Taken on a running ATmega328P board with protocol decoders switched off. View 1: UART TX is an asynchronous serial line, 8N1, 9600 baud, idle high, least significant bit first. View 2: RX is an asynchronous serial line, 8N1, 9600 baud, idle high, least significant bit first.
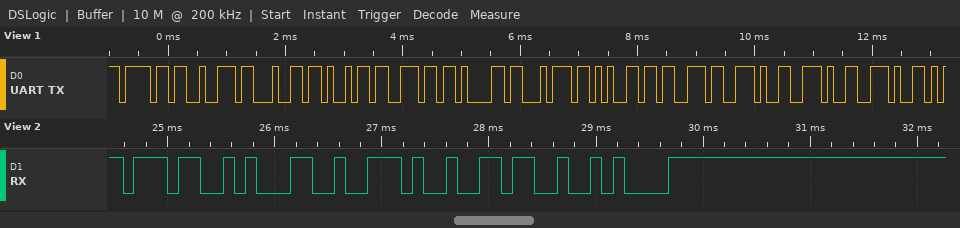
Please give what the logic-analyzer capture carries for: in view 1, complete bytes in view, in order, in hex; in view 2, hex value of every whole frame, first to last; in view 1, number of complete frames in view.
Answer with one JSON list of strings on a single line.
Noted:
["6F 72 64 69 6E 61 74 65 73 2E 2E 2E", "37 31 2E 36 0A", "12"]
